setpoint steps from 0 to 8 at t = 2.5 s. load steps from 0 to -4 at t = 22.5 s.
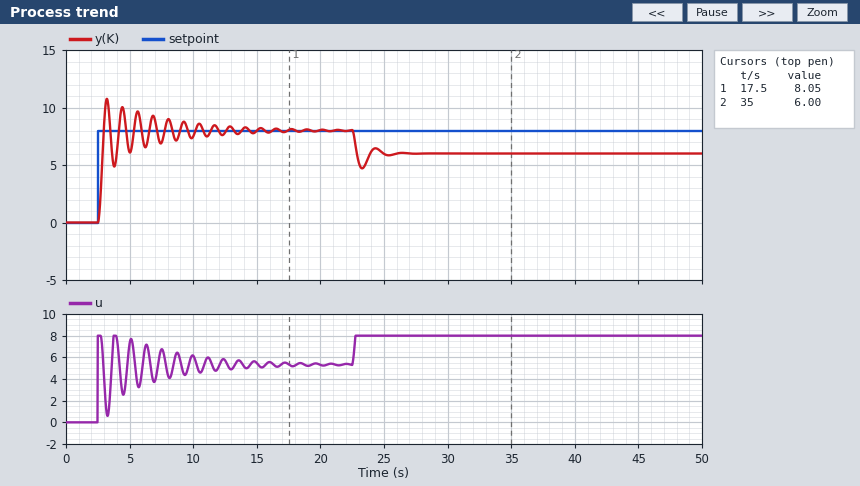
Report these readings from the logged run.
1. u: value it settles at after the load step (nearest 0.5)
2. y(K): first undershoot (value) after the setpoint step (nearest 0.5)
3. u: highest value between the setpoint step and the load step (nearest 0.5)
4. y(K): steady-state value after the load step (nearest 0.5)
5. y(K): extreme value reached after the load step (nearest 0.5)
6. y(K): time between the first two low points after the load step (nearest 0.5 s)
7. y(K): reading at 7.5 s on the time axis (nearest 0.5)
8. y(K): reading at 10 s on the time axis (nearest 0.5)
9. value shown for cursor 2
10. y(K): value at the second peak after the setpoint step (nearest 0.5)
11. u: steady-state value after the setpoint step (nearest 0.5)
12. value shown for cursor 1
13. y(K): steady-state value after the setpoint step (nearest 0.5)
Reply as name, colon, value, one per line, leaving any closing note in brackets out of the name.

u: value it settles at after the load step: 8.0
y(K): first undershoot (value) after the setpoint step: 5.0
u: highest value between the setpoint step and the load step: 8.0
y(K): steady-state value after the load step: 6.0
y(K): extreme value reached after the load step: 4.5
y(K): time between the first two low points after the load step: 2.0 s
y(K): reading at 7.5 s on the time axis: 7.0
y(K): reading at 10 s on the time axis: 7.5
value shown for cursor 2: 6.00
y(K): value at the second peak after the setpoint step: 10.0
u: steady-state value after the setpoint step: 5.5
value shown for cursor 1: 8.05
y(K): steady-state value after the setpoint step: 8.0
